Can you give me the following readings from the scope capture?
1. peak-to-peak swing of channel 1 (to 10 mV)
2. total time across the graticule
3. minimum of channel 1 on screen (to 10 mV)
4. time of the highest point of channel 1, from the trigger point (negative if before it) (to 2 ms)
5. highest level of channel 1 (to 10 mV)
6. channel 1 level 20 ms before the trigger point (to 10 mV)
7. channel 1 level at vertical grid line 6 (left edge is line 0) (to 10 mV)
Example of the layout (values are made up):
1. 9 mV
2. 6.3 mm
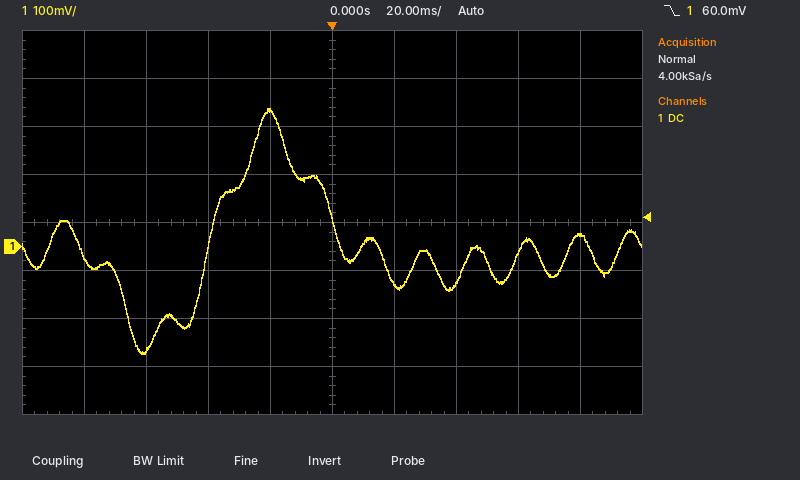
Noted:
1. 510 mV
2. 200 ms
3. -220 mV
4. -20 ms
5. 290 mV
6. 280 mV
7. -80 mV
